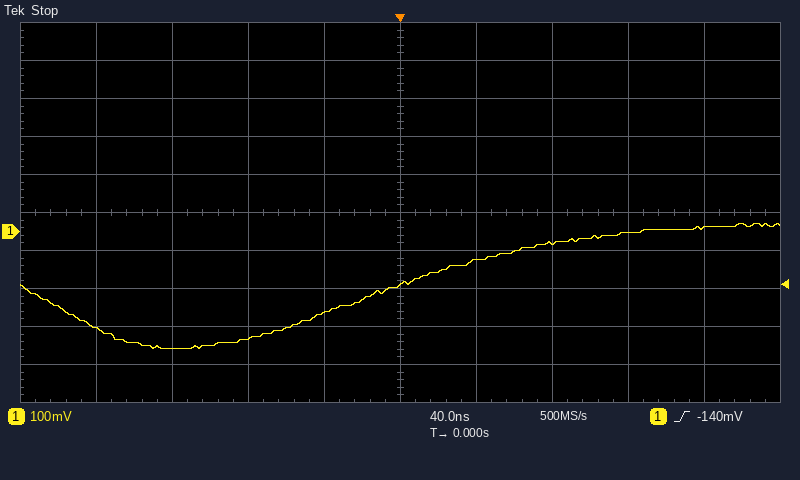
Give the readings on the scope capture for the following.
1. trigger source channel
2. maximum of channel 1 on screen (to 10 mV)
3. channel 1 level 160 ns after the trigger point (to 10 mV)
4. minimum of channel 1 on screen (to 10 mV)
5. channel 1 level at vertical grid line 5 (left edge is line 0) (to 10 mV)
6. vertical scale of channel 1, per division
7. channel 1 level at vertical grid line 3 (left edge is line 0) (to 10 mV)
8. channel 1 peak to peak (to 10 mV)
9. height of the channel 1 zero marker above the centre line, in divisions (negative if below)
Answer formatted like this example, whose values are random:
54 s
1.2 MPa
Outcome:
channel 1
20 mV
10 mV
-310 mV
-140 mV
100 mV
-280 mV
330 mV
-0.5 div
